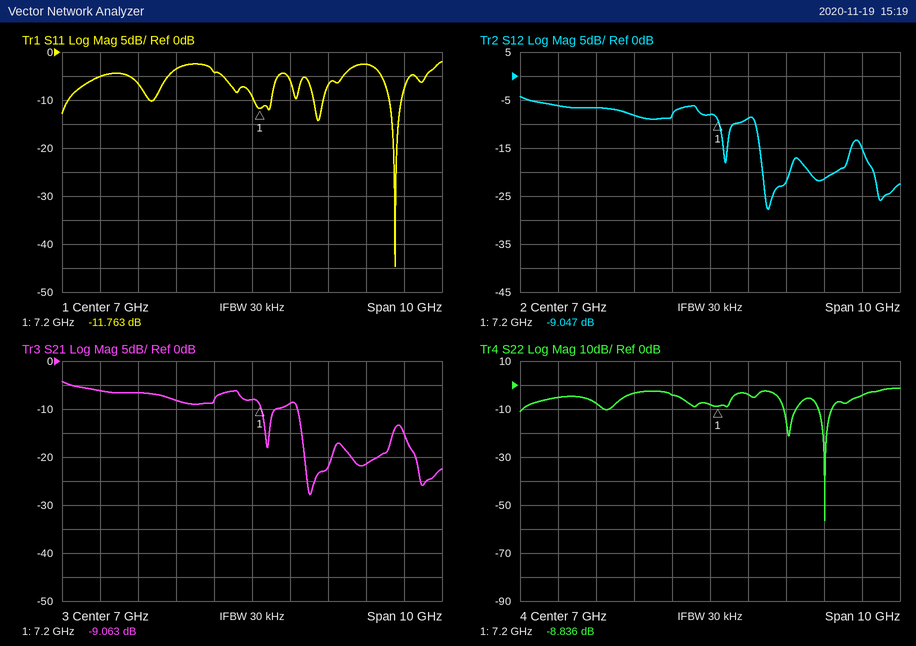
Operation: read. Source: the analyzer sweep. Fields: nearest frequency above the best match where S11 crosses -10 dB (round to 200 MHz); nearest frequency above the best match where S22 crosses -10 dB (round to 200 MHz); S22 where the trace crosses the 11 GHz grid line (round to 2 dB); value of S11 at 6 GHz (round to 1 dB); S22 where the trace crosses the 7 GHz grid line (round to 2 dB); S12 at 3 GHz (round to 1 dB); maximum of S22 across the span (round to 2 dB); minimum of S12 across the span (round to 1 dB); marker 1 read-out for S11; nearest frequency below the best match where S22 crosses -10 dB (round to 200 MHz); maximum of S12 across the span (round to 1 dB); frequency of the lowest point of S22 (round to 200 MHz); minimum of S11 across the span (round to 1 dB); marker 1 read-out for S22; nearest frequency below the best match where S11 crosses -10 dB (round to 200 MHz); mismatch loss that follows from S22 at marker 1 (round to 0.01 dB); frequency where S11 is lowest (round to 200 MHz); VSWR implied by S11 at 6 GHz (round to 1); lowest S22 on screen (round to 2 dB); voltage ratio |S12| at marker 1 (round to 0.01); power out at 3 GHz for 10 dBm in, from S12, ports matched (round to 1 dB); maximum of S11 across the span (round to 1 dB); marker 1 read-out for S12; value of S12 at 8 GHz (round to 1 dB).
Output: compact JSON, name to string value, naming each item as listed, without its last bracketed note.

{"nearest frequency above the best match where S11 crosses -10 dB": "11.0 GHz", "nearest frequency above the best match where S22 crosses -10 dB": "10.2 GHz", "S22 where the trace crosses the 11 GHz grid line": "-4 dB", "value of S11 at 6 GHz": "-4 dB", "S22 where the trace crosses the 7 GHz grid line": "-8 dB", "S12 at 3 GHz": "-6 dB", "maximum of S22 across the span": "-2 dB", "minimum of S12 across the span": "-28 dB", "marker 1 read-out for S11": "-11.763 dB", "nearest frequency below the best match where S22 crosses -10 dB": "9.8 GHz", "maximum of S12 across the span": "-4 dB", "frequency of the lowest point of S22": "10.0 GHz", "minimum of S11 across the span": "-45 dB", "marker 1 read-out for S22": "-8.836 dB", "nearest frequency below the best match where S11 crosses -10 dB": "10.6 GHz", "mismatch loss that follows from S22 at marker 1": "0.61 dB", "frequency where S11 is lowest": "10.8 GHz", "VSWR implied by S11 at 6 GHz": "4", "lowest S22 on screen": "-56 dB", "voltage ratio |S12| at marker 1": "0.35", "power out at 3 GHz for 10 dBm in, from S12, ports matched": "4 dBm", "maximum of S11 across the span": "-2 dB", "marker 1 read-out for S12": "-9.047 dB", "value of S12 at 8 GHz": "-9 dB"}
